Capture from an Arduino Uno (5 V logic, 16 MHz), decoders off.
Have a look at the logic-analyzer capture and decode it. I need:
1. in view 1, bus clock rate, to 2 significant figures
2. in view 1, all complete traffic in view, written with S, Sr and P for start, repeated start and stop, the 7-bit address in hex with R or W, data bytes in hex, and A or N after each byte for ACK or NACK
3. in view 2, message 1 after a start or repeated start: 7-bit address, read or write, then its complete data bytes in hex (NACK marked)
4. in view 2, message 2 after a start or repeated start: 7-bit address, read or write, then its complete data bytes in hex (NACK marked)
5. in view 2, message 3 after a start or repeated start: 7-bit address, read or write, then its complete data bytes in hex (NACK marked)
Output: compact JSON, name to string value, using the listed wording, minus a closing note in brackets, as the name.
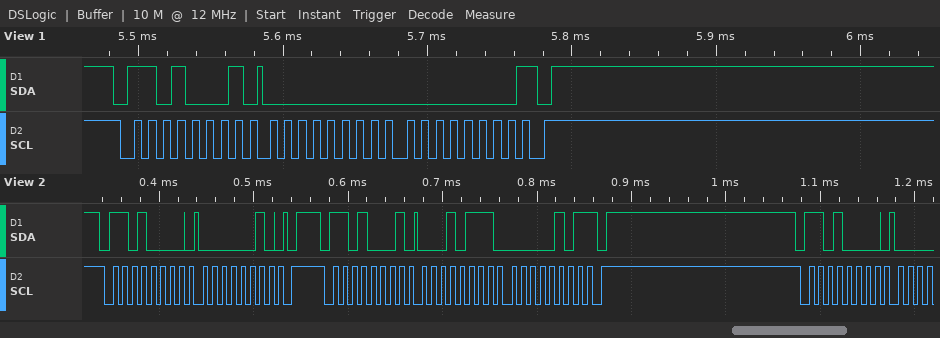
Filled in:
{"in view 1, bus clock rate, to 2 significant figures": "100 kHz", "in view 1, all complete traffic in view, written with S, Sr and P for start, repeated start and stop, the 7-bit address in hex with R or W, data bytes in hex, and A or N after each byte for ACK or NACK": "S 68R A 00 A 00 N P", "in view 2, message 1 after a start or repeated start: 7-bit address, read or write, then its complete data bytes in hex": "0x68 write: 02", "in view 2, message 2 after a start or repeated start: 7-bit address, read or write, then its complete data bytes in hex": "0x68 read: 17 05 NACK", "in view 2, message 3 after a start or repeated start: 7-bit address, read or write, then its complete data bytes in hex": "0x68 write"}
